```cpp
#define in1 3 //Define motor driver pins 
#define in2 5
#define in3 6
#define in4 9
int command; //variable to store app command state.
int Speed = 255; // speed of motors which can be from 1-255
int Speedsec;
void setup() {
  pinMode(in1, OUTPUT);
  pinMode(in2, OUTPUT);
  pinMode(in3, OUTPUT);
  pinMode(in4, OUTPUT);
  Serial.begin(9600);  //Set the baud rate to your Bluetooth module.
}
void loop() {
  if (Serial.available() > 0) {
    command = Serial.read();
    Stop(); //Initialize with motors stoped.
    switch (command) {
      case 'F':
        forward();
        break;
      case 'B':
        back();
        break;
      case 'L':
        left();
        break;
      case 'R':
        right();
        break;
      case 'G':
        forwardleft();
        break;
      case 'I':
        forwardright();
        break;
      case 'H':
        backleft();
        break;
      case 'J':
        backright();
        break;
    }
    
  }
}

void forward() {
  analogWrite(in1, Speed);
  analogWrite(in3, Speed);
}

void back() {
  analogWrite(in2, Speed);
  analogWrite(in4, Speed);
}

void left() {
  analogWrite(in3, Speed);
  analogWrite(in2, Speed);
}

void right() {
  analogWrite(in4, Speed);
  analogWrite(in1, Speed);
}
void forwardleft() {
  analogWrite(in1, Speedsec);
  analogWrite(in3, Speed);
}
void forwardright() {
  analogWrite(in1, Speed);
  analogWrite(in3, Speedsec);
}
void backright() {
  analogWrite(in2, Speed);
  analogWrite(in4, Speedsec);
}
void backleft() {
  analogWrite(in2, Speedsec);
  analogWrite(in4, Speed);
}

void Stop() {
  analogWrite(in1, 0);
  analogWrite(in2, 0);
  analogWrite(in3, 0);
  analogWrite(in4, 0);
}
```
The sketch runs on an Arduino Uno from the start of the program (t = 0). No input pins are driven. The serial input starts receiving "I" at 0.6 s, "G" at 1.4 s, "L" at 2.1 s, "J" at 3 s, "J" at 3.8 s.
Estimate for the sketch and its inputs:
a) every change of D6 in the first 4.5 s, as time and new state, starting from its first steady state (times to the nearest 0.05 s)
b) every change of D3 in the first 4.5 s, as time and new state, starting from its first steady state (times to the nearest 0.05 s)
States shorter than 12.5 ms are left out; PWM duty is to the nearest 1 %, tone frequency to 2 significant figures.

0 s low; 1.4 s high; 3 s low
0 s low; 0.6 s high; 1.4 s low
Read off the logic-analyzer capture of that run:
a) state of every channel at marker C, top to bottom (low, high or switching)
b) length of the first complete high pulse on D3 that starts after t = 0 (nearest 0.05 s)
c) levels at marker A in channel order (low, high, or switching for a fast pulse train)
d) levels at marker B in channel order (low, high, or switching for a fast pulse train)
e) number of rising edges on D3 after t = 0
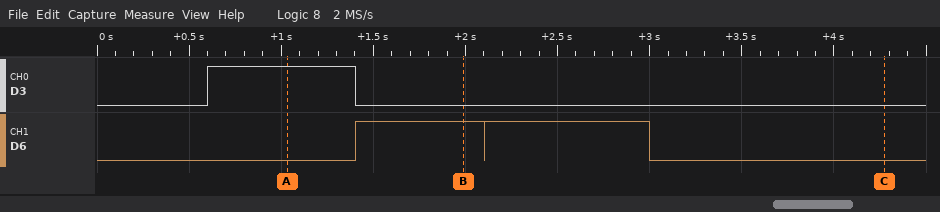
D3 low, D6 low
0.80 s
D3 high, D6 low
D3 low, D6 high
1
